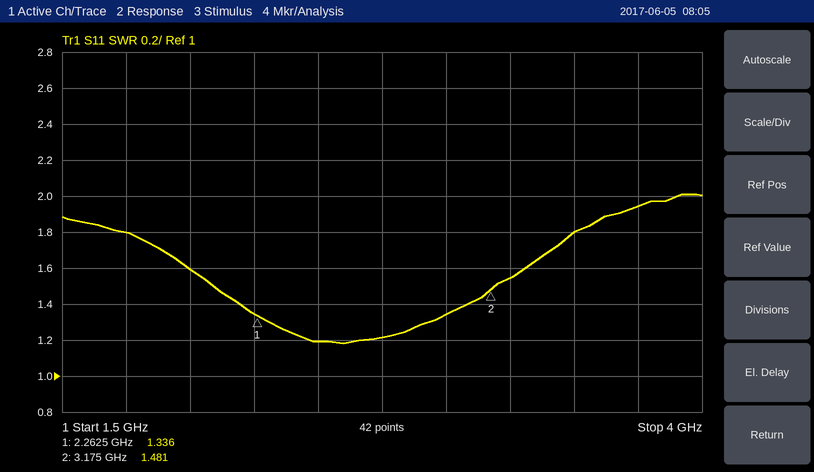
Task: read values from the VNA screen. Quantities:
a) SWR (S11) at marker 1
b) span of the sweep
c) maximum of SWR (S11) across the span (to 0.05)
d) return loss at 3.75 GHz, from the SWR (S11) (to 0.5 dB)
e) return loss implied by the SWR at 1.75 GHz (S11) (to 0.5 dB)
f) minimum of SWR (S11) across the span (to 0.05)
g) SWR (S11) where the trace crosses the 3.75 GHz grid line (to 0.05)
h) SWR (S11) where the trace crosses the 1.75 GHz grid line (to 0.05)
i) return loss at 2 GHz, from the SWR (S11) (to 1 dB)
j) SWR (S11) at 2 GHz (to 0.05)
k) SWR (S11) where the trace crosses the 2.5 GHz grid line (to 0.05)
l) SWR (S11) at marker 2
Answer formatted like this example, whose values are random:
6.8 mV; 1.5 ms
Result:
1.336; 2.5 GHz; 2.00; 10.0 dB; 11.0 dB; 1.20; 1.95; 1.80; 13 dB; 1.60; 1.20; 1.481
